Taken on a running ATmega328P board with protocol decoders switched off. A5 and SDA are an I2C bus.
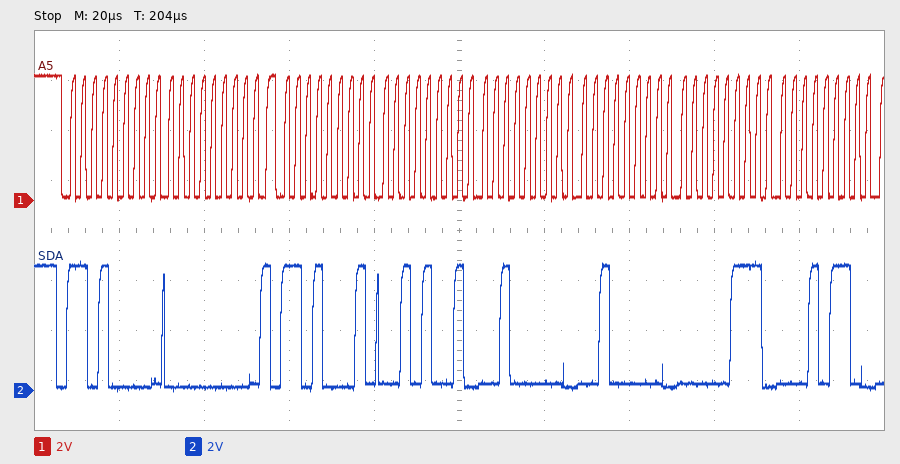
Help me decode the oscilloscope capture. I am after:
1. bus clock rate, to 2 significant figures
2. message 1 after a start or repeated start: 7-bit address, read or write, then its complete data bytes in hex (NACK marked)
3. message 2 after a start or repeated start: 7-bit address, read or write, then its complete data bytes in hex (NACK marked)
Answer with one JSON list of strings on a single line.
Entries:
["400 kHz", "0x68 write: 00", "0x68 read: 29 20 20 07 16"]
